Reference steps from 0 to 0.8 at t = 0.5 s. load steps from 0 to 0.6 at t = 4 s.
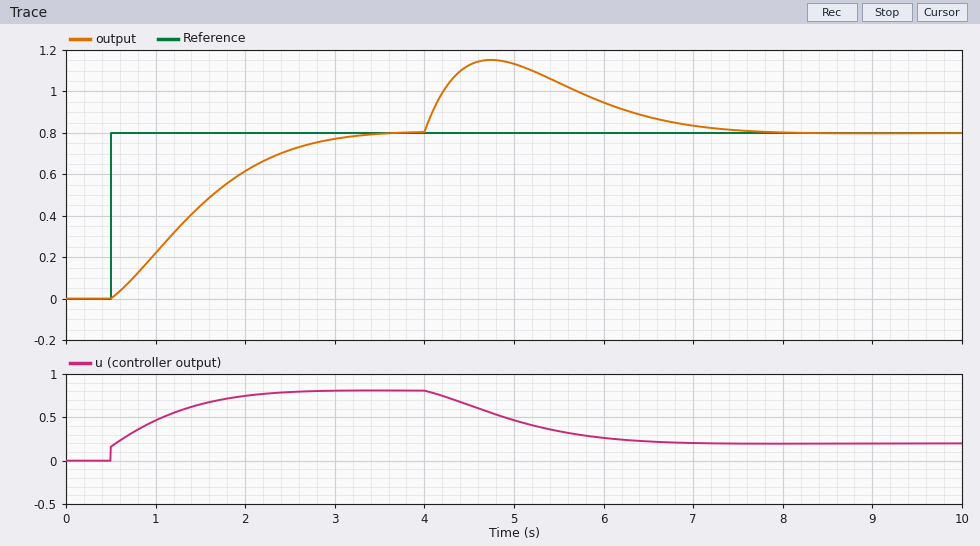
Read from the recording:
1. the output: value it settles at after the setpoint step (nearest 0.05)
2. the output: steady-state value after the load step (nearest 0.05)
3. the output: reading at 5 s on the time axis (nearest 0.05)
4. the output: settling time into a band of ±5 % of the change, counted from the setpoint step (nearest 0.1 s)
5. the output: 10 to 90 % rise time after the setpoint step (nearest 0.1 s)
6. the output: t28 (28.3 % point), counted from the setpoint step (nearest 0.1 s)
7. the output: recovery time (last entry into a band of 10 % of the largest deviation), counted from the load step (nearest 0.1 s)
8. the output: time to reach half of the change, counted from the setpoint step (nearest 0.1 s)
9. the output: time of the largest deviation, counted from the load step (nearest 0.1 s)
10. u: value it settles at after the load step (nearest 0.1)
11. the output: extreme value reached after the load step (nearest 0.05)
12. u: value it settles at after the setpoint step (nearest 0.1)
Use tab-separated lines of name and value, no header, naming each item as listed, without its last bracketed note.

the output: value it settles at after the setpoint step	0.80
the output: steady-state value after the load step	0.80
the output: reading at 5 s on the time axis	1.15
the output: settling time into a band of ±5 % of the change, counted from the setpoint step	2.4 s
the output: 10 to 90 % rise time after the setpoint step	1.8 s
the output: t28 (28.3 % point), counted from the setpoint step	0.5 s
the output: recovery time (last entry into a band of 10 % of the largest deviation), counted from the load step	3.0 s
the output: time to reach half of the change, counted from the setpoint step	0.9 s
the output: time of the largest deviation, counted from the load step	0.7 s
u: value it settles at after the load step	0.2
the output: extreme value reached after the load step	1.15
u: value it settles at after the setpoint step	0.8
